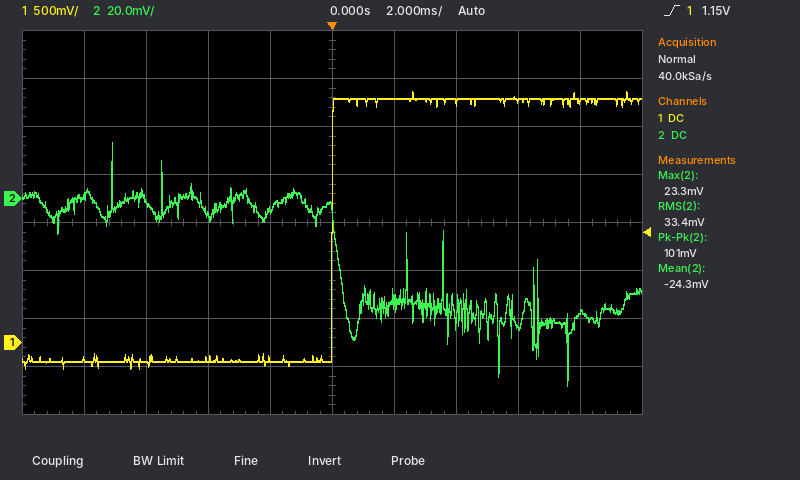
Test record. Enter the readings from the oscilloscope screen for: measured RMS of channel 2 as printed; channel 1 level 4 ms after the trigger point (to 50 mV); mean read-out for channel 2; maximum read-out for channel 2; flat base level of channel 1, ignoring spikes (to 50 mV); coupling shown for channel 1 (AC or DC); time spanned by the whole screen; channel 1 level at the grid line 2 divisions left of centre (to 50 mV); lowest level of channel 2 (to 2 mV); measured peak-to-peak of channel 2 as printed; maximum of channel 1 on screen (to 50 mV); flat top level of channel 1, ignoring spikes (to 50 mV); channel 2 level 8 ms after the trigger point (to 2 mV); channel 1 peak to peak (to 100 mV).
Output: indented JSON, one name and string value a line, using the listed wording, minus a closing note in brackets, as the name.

{
  "measured RMS of channel 2 as printed": "33.4 mV",
  "channel 1 level 4 ms after the trigger point": "2.50 V",
  "mean read-out for channel 2": "-24.3 mV",
  "maximum read-out for channel 2": "23.3 mV",
  "flat base level of channel 1, ignoring spikes": "-200 mV",
  "coupling shown for channel 1": "DC",
  "time spanned by the whole screen": "20 ms",
  "channel 1 level at the grid line 2 divisions left of centre": "-150 mV",
  "lowest level of channel 2": "-78 mV",
  "measured peak-to-peak of channel 2 as printed": "101 mV",
  "maximum of channel 1 on screen": "2.60 V",
  "flat top level of channel 1, ignoring spikes": "2.55 V",
  "channel 2 level 8 ms after the trigger point": "-48 mV",
  "channel 1 peak to peak": "2.90 V"
}
